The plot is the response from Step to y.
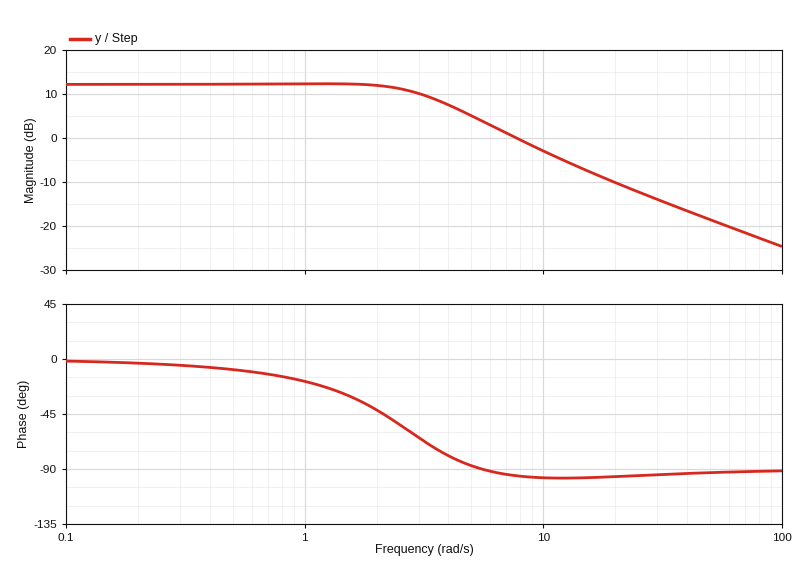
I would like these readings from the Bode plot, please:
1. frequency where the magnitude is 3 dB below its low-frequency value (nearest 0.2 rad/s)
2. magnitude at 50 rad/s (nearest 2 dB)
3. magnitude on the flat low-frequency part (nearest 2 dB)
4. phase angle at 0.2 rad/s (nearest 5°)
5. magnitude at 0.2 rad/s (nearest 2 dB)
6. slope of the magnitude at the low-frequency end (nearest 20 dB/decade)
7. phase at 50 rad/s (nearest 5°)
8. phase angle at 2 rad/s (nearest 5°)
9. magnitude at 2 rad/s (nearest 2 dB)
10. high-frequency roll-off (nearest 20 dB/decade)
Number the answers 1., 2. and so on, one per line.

1. 3.4 rad/s
2. -18 dB
3. 12 dB
4. -5°
5. 12 dB
6. 0 dB/decade
7. -95°
8. -40°
9. 12 dB
10. -20 dB/decade
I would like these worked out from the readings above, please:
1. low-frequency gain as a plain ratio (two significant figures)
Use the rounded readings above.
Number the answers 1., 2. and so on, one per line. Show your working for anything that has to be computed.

1. 10^(12 / 20) = 4.0
